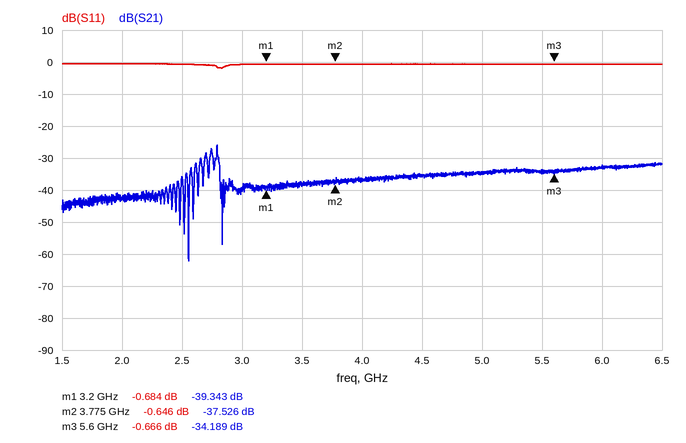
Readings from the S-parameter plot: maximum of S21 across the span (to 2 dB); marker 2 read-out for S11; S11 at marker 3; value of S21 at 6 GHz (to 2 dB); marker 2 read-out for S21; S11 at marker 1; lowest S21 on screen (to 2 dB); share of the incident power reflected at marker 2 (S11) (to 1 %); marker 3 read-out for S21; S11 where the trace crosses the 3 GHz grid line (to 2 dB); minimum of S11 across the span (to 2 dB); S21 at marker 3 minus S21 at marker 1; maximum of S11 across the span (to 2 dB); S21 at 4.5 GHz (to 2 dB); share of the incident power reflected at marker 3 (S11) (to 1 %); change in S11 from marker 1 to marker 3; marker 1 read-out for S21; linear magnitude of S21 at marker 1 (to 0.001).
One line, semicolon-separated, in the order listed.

-26 dB; -0.646 dB; -0.666 dB; -32 dB; -37.526 dB; -0.684 dB; -62 dB; 86 %; -34.189 dB; 0 dB; -2 dB; 5.154 dB; 0 dB; -36 dB; 86 %; 0.018 dB; -39.343 dB; 0.011
